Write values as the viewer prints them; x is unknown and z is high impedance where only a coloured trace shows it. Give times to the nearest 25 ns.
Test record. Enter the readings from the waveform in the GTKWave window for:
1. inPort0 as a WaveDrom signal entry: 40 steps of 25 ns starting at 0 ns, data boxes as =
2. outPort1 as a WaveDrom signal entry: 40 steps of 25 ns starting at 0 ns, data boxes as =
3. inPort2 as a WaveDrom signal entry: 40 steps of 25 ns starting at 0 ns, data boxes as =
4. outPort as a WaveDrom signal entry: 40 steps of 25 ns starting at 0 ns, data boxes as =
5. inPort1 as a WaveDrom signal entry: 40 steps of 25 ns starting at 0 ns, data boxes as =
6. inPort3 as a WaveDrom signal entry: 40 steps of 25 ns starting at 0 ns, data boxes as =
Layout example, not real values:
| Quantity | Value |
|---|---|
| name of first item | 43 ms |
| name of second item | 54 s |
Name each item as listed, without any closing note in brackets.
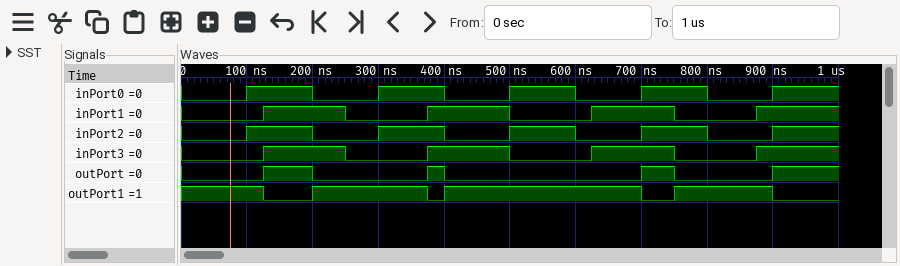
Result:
| Quantity | Value |
|---|---|
| inPort0 as a WaveDrom signal entry: 40 steps of 25 ns starting at 0 ns, data boxes as = | {name: 'inPort0', wave: '0...1...0...1...0...1...0...1...0...1...'} |
| outPort1 as a WaveDrom signal entry: 40 steps of 25 ns starting at 0 ns, data boxes as = | {name: 'outPort1', wave: '1....0..1......01...........0.1.....0...'} |
| inPort2 as a WaveDrom signal entry: 40 steps of 25 ns starting at 0 ns, data boxes as = | {name: 'inPort2', wave: '0...1...0...1...0...1...0...1...0...1...'} |
| outPort as a WaveDrom signal entry: 40 steps of 25 ns starting at 0 ns, data boxes as = | {name: 'outPort', wave: '0....1..0......10...........1.0.....1...'} |
| inPort1 as a WaveDrom signal entry: 40 steps of 25 ns starting at 0 ns, data boxes as = | {name: 'inPort1', wave: '0....1....0....1....0....1....0....1....'} |
| inPort3 as a WaveDrom signal entry: 40 steps of 25 ns starting at 0 ns, data boxes as = | {name: 'inPort3', wave: '0....1....0....1....0....1....0....1....'} |
